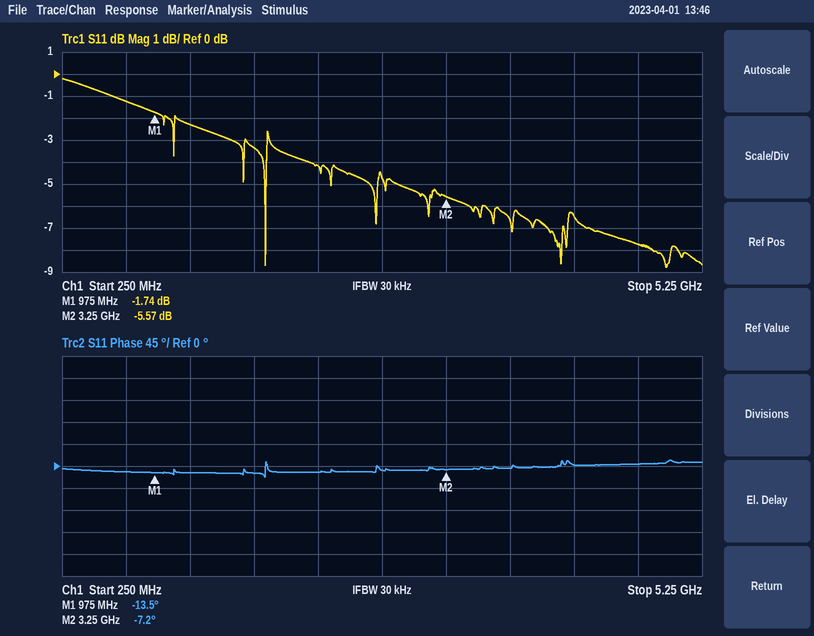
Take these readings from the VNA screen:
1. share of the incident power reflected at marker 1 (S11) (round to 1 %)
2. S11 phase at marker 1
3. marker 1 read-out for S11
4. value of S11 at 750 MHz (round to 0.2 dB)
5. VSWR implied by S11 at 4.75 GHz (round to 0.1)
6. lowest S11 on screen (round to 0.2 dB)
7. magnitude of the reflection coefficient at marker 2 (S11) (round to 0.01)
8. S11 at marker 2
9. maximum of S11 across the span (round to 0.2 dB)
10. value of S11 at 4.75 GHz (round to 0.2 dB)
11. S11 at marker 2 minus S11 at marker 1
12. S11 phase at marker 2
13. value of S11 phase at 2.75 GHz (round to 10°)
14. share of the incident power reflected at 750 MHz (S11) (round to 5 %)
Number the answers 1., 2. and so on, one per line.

1. 67 %
2. -13.5°
3. -1.74 dB
4. -1.2 dB
5. 2.4
6. -8.8 dB
7. 0.53
8. -5.57 dB
9. -0.2 dB
10. -7.8 dB
11. -3.83 dB
12. -7.2°
13. -10°
14. 75 %
